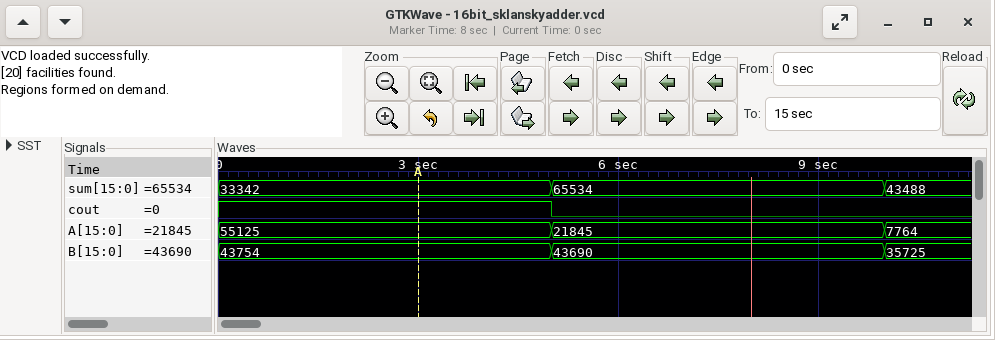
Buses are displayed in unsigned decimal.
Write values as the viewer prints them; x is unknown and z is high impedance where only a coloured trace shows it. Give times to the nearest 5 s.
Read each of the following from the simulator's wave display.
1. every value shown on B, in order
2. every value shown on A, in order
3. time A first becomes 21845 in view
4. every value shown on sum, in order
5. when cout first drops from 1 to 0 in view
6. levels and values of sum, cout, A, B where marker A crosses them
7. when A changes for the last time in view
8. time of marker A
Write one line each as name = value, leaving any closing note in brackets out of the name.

every value shown on B, in order = 43754, 43690, 35725
every value shown on A, in order = 55125, 21845, 7764
time A first becomes 21845 in view = 5 s
every value shown on sum, in order = 33342, 65534, 43488
when cout first drops from 1 to 0 in view = 5 s
levels and values of sum, cout, A, B where marker A crosses them = sum=33342, cout=1, A=55125, B=43754
when A changes for the last time in view = 10 s
time of marker A = 5 s
